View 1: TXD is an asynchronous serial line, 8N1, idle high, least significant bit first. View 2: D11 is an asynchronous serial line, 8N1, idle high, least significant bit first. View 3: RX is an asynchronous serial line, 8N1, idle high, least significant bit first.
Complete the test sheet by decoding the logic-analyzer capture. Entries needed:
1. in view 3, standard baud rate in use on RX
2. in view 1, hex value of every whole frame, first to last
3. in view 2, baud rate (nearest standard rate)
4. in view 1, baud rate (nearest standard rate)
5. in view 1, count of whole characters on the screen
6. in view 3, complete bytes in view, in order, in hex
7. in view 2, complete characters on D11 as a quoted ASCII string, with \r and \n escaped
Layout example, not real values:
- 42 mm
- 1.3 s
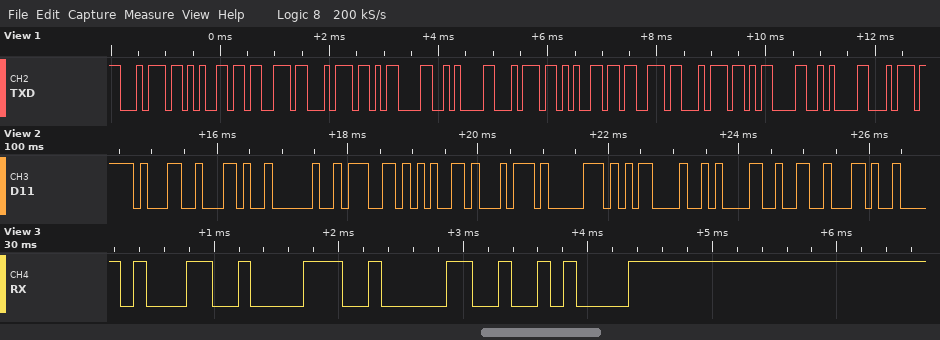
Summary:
- 9600 baud
- 74 65 73 74 0D 0A 74 65 73 74 0D 0A 74
- 9600 baud
- 9600 baud
- 13
- 0x31 0x38 0x30 0x0A
- "1, getp\r\n2,"
